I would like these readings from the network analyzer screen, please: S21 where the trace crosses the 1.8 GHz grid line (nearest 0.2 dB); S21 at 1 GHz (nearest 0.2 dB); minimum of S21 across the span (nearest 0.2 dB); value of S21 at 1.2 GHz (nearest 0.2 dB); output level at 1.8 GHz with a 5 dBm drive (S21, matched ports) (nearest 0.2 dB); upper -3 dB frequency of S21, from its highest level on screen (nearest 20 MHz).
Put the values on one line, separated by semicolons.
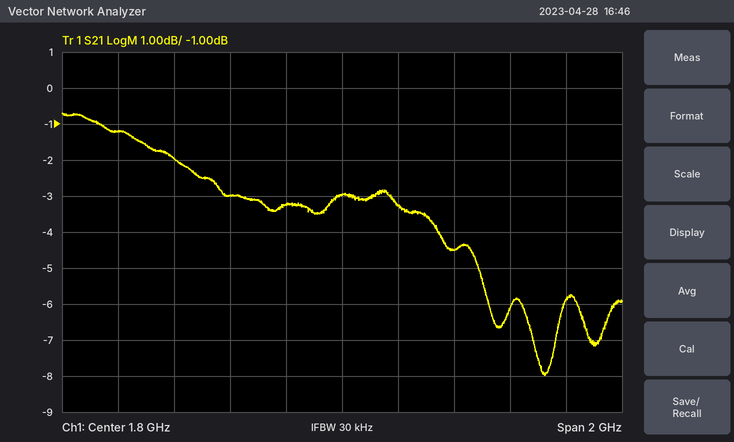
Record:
-3.0 dB; -1.2 dB; -8.0 dB; -2.0 dB; 2.0 dBm; 2.12 GHz
